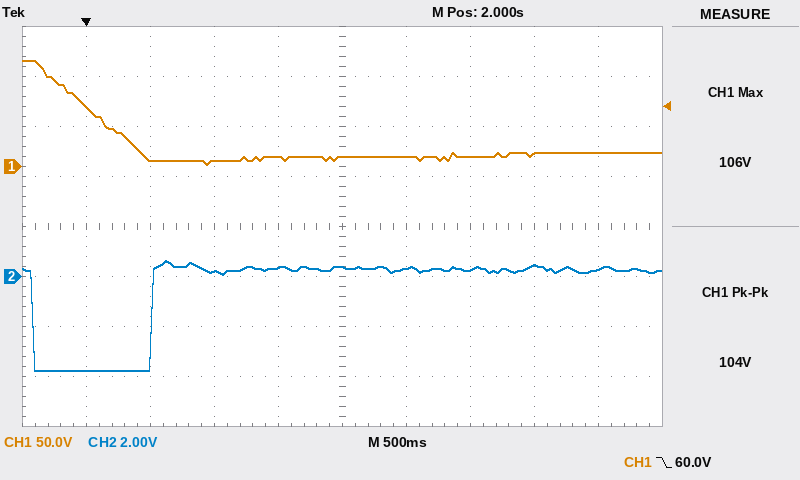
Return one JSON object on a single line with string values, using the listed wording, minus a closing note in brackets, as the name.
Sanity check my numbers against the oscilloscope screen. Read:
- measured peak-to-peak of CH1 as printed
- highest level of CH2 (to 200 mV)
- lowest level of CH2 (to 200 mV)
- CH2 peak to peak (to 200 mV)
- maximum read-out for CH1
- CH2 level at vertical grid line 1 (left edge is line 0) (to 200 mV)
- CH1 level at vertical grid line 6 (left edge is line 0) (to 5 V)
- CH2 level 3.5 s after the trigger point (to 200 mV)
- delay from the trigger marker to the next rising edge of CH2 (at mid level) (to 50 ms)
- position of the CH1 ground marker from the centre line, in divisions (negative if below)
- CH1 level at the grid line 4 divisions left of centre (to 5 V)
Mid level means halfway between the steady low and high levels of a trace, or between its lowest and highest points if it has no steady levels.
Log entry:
{"measured peak-to-peak of CH1 as printed": "104 V", "highest level of CH2": "600 mV", "lowest level of CH2": "-3.8 V", "CH2 peak to peak": "4.4 V", "maximum read-out for CH1": "106 V", "CH2 level at vertical grid line 1 (left edge is line 0)": "-3.8 V", "CH1 level at vertical grid line 6 (left edge is line 0)": "10 V", "CH2 level 3.5 s after the trigger point": "400 mV", "delay from the trigger marker to the next rising edge of CH2 (at mid level)": "500 ms", "position of the CH1 ground marker from the centre line, in divisions": "+1.2 div", "CH1 level at the grid line 4 divisions left of centre": "60 V"}
